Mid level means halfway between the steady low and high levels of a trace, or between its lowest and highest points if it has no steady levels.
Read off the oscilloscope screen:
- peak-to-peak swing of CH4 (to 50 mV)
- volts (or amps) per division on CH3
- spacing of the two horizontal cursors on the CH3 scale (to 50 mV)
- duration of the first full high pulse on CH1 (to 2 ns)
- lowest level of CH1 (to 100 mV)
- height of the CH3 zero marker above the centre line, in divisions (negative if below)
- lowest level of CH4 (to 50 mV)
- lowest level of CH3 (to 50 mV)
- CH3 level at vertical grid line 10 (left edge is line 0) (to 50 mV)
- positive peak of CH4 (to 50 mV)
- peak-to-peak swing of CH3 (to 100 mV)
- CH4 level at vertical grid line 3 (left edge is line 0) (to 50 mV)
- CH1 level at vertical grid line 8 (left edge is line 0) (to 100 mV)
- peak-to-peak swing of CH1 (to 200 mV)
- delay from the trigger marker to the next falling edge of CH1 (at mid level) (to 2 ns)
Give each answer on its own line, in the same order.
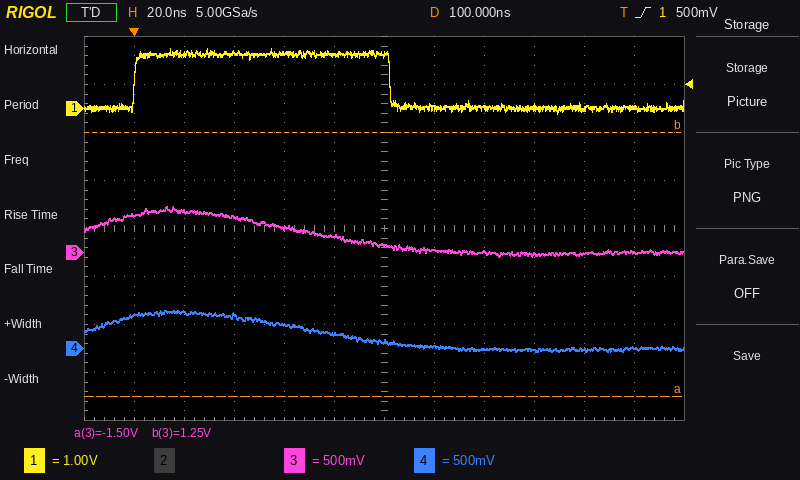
450 mV
500 mV
2.75 V
102 ns
-100 mV
-0.5 div
-50 mV
-50 mV
0 mV
400 mV
500 mV
350 mV
0.0 V
1.4 V
102 ns
